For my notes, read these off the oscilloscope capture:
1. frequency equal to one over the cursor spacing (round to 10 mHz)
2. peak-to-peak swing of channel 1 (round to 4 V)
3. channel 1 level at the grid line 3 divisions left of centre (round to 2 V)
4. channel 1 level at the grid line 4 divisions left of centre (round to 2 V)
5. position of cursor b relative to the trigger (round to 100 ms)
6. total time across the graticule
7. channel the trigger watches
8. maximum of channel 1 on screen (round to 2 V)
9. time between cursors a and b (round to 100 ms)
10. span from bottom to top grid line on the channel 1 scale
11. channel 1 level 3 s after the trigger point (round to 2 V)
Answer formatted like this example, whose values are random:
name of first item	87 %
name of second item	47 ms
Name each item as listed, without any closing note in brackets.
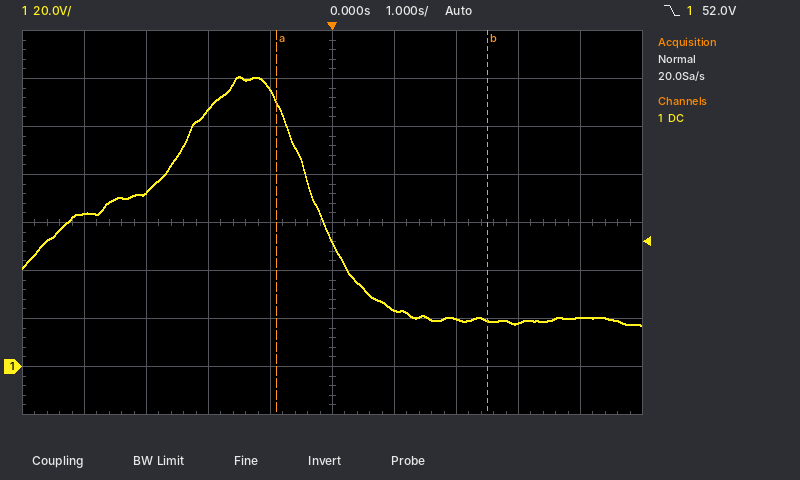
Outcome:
frequency equal to one over the cursor spacing	290 mHz
peak-to-peak swing of channel 1	104 V
channel 1 level at the grid line 3 divisions left of centre	72 V
channel 1 level at the grid line 4 divisions left of centre	64 V
position of cursor b relative to the trigger	+2.5 s
total time across the graticule	10 s
channel the trigger watches	channel 1
maximum of channel 1 on screen	120 V
time between cursors a and b	3.4 s
span from bottom to top grid line on the channel 1 scale	160 V
channel 1 level 3 s after the trigger point	18 V
